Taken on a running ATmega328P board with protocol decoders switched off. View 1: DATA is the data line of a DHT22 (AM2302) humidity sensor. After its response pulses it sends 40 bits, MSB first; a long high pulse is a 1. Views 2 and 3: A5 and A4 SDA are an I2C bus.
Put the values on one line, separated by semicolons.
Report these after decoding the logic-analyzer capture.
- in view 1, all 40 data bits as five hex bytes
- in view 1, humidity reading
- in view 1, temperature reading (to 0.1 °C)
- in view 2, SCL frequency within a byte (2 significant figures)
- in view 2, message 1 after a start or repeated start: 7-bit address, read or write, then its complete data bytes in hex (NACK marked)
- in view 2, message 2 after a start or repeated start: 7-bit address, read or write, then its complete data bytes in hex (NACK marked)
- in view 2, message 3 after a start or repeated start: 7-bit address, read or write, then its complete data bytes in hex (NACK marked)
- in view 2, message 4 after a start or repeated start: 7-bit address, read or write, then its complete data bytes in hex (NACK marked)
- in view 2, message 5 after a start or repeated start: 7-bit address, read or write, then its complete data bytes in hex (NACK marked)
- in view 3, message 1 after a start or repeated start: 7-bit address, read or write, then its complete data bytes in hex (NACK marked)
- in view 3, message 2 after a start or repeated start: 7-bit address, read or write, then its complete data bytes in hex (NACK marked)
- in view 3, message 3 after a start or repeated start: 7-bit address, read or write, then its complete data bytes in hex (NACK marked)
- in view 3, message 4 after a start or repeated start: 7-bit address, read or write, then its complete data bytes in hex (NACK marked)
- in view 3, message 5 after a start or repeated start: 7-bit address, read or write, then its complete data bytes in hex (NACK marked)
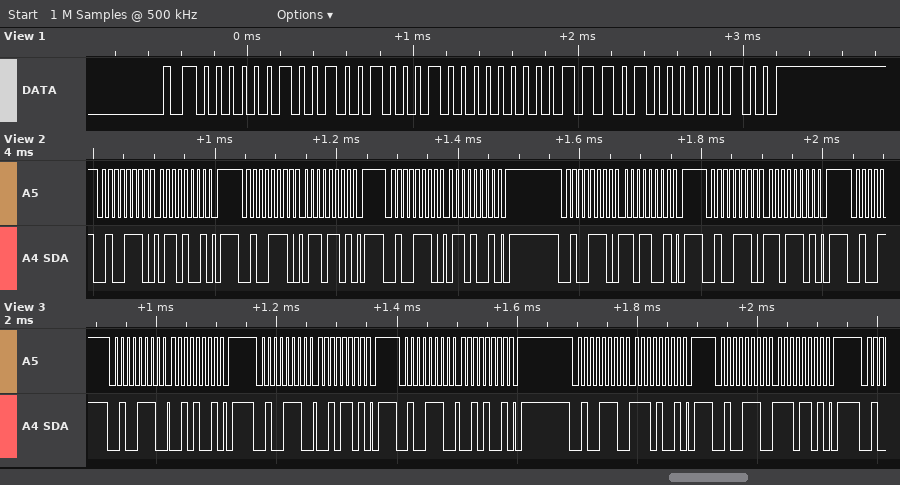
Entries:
02 48 80 3A 04; 58.4 %; -5.8 °C; 100 kHz; 0x27 write: 69; 0x27 write: 6D; 0x27 write: 69; 0x27 write: D9; 0x27 write: DD; 0x27 write: 29; 0x27 write: 2D; 0x27 write: 29; 0x27 write: E9; 0x27 write: ED
